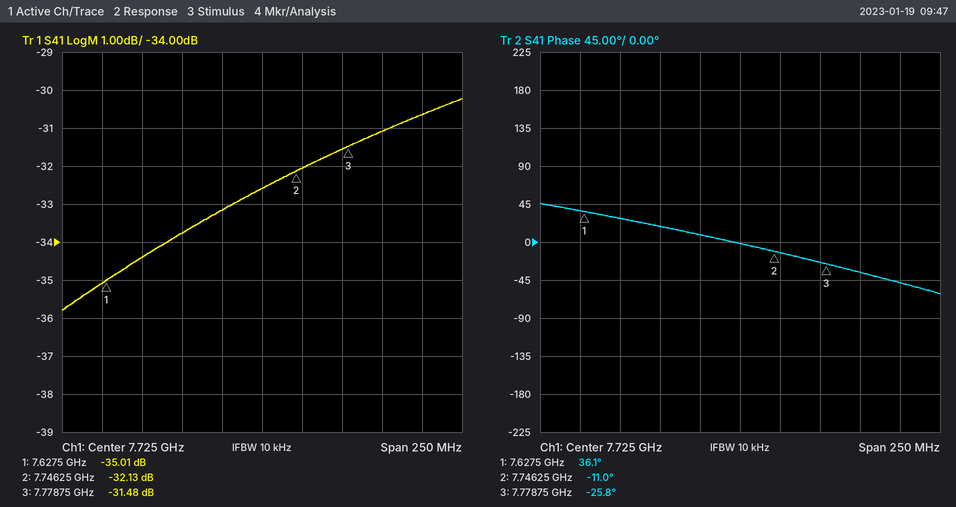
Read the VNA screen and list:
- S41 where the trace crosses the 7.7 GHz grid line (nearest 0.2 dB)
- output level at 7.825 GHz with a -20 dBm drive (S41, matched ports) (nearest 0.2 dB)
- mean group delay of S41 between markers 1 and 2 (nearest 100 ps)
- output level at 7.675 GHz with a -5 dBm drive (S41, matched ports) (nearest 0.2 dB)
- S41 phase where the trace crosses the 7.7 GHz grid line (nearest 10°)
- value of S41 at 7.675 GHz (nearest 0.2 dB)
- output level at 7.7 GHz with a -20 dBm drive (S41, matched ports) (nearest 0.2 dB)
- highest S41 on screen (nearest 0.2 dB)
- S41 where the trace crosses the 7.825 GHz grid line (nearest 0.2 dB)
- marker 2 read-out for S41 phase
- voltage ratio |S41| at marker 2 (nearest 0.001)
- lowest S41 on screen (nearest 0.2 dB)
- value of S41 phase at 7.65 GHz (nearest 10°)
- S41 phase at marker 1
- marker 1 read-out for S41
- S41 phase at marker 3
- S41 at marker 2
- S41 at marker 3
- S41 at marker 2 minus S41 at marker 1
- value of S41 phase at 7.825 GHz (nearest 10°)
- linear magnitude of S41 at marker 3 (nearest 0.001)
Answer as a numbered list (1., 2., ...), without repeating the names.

1. -33.2 dB
2. -50.6 dBm
3. 1.1 ns
4. -38.8 dBm
5. 10°
6. -33.8 dB
7. -53.2 dBm
8. -30.2 dB
9. -30.6 dB
10. -11.0°
11. 0.025
12. -35.8 dB
13. 30°
14. 36.1°
15. -35.01 dB
16. -25.8°
17. -32.13 dB
18. -31.48 dB
19. 2.88 dB
20. -50°
21. 0.027
